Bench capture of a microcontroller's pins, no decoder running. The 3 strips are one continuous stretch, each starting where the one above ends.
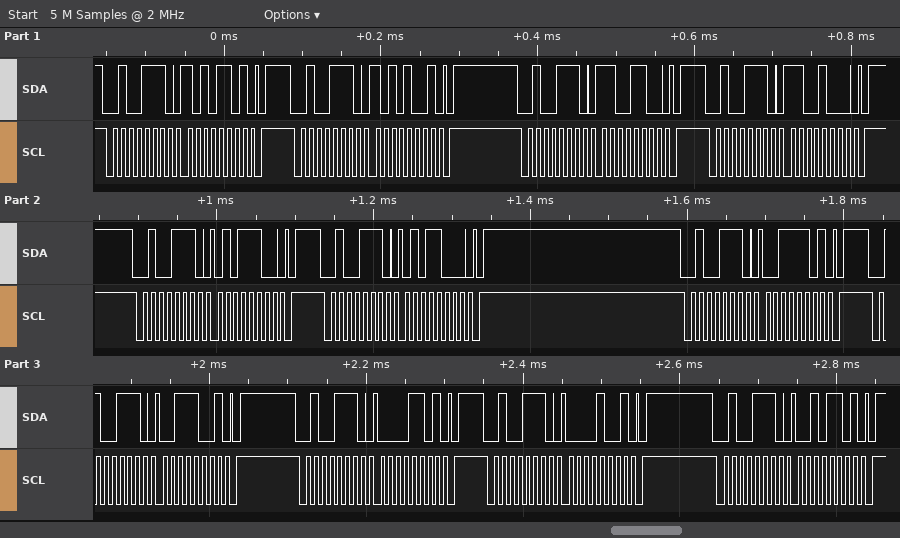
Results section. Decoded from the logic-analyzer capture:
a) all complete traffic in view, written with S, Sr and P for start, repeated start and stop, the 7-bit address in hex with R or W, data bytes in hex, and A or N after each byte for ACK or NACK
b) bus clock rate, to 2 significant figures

S 27W A AD A P S 27W A A9 A P S 27W A CC A P S 27W A C8 A P S 27W A 5C A P S 27W A 58 A P S 27W A 3D A P S 27W A 39 A P S 27W A 0D A P S 27W A 09 A P S 27W A 2D A P
100 kHz
